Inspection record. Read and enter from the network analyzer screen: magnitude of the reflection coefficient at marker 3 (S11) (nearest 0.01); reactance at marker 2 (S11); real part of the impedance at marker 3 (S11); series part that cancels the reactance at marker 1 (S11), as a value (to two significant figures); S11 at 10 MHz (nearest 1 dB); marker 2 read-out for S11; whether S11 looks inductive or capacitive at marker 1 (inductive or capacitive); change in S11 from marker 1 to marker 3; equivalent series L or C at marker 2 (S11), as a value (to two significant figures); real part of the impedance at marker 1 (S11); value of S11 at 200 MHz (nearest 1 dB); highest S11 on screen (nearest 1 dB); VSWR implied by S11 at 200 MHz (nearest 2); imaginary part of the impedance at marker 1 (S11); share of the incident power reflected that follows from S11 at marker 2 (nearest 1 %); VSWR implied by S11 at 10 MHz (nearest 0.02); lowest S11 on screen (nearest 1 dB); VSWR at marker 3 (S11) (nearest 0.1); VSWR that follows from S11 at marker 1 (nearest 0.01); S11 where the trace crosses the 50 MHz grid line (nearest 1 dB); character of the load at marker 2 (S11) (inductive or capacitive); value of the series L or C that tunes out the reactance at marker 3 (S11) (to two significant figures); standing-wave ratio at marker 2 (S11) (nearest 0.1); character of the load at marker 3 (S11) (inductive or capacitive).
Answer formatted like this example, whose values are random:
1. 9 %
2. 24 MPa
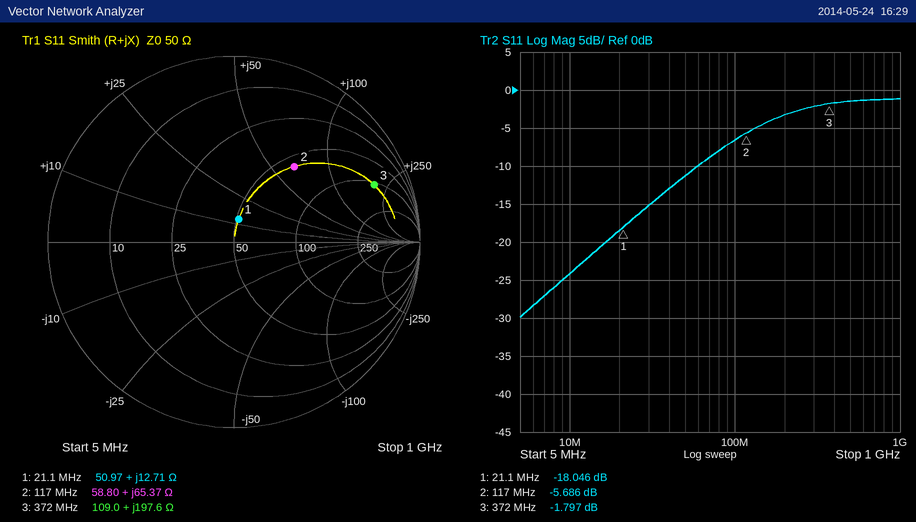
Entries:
1. 0.81
2. +65.37 Ω
3. 109.0 Ω
4. 590 pF
5. -24 dB
6. -5.686 dB
7. inductive
8. 16.249 dB
9. 89 nH
10. 50.97 Ω
11. -3 dB
12. -1 dB
13. 6
14. +12.71 Ω
15. 27 %
16. 1.14
17. -30 dB
18. 9.7
19. 1.29
20. -11 dB
21. inductive
22. 2.2 pF
23. 3.2
24. inductive
